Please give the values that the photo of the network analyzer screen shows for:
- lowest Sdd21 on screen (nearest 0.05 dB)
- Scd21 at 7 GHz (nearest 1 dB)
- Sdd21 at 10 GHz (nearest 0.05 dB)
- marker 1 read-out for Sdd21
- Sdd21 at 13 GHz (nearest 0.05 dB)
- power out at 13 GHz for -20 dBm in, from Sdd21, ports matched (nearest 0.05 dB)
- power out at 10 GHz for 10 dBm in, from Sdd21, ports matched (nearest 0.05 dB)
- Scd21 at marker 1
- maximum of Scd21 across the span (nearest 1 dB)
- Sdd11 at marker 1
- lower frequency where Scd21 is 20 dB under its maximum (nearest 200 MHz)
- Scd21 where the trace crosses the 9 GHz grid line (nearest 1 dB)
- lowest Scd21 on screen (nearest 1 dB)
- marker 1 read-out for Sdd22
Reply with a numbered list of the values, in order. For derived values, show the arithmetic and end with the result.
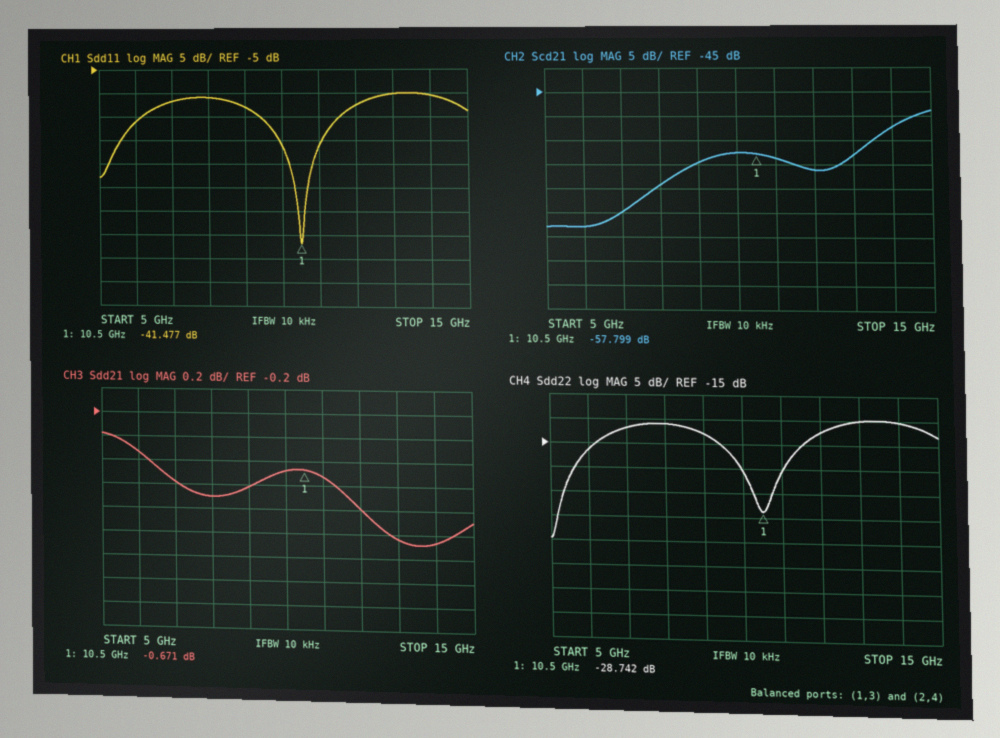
1. -1.30 dB
2. -70 dB
3. -0.70 dB
4. -0.671 dB
5. -1.25 dB
6. -20 dBm + (-1.25 dB) = -21.25 dBm
7. 10 dBm + (-0.70 dB) = 9.30 dBm
8. -57.799 dB
9. -49 dB
10. -41.477 dB
11. 7.2 GHz
12. -60 dB
13. -73 dB
14. -28.742 dB
